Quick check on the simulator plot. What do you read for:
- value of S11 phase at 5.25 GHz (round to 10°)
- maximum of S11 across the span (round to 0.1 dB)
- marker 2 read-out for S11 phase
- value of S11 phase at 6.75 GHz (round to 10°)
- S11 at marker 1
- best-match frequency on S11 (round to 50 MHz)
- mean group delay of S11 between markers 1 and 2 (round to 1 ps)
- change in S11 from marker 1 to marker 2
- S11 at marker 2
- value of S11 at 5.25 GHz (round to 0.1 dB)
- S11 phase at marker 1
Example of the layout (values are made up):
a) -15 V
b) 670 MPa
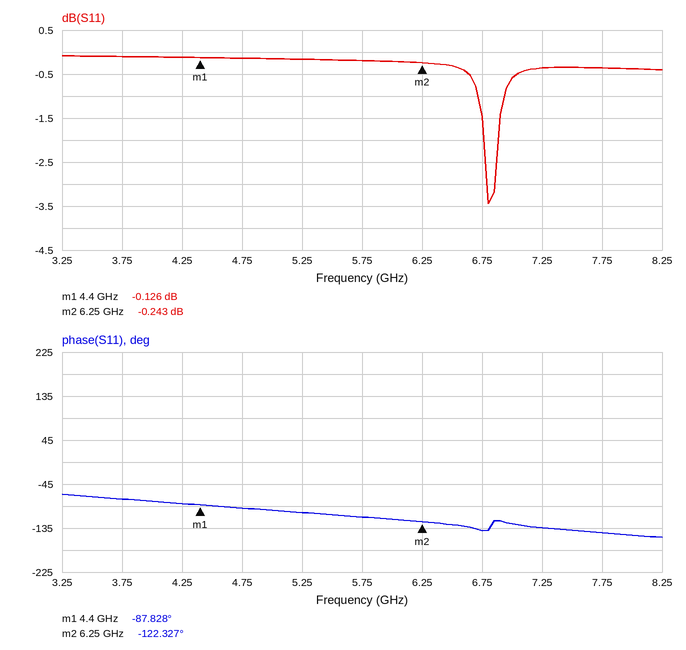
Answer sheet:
a) -100°
b) -0.1 dB
c) -122.327°
d) -140°
e) -0.126 dB
f) 6.80 GHz
g) 52 ps
h) -0.117 dB
i) -0.243 dB
j) -0.2 dB
k) -87.828°
